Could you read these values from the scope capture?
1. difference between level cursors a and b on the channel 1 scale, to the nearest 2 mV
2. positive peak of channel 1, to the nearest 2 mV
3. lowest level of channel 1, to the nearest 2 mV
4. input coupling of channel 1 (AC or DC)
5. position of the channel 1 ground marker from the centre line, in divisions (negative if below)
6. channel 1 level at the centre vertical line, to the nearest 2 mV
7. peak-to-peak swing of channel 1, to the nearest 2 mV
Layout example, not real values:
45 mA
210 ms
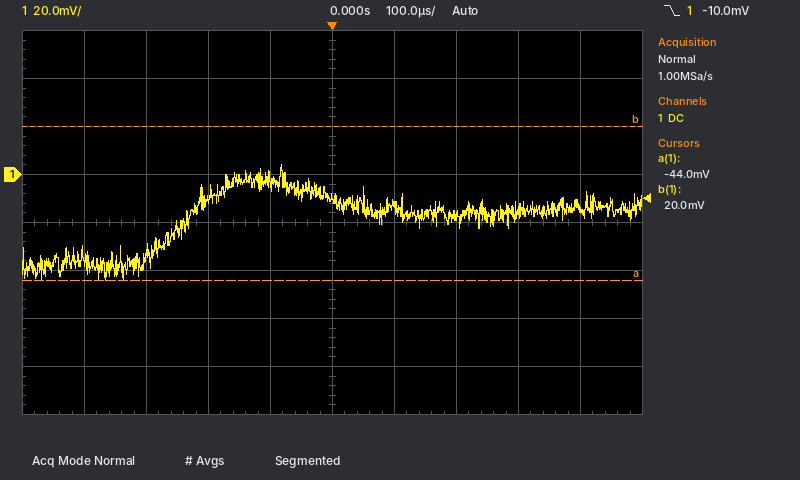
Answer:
64 mV
4 mV
-44 mV
DC
+1.0 div
-10 mV
48 mV
